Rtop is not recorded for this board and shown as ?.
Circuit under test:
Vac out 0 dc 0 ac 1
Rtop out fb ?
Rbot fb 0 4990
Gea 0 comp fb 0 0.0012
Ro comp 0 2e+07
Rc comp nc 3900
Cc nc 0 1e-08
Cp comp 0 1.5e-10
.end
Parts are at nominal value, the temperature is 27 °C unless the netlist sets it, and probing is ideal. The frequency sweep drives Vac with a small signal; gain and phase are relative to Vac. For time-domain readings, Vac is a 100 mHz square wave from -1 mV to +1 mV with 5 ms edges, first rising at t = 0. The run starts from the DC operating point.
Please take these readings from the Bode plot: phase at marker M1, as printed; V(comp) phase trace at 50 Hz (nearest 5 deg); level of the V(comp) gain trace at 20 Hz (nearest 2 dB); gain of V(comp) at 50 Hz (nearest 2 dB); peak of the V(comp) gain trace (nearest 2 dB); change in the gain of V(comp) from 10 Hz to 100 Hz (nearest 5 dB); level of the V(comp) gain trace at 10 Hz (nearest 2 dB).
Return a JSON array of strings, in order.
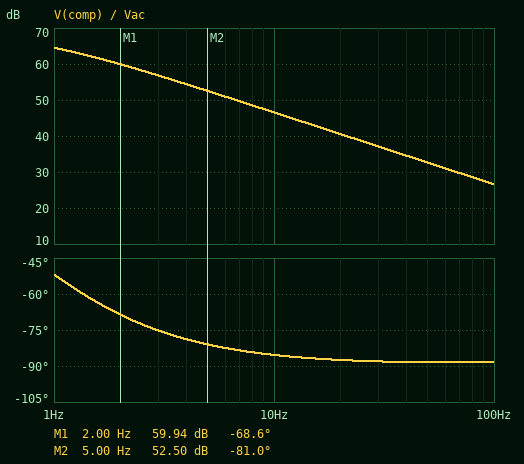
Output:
["-68.6 deg", "-90 deg", "40 dB", "32 dB", "64 dB", "-20 dB", "46 dB"]
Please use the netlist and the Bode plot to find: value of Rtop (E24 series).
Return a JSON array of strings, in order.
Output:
["39 kΩ"]
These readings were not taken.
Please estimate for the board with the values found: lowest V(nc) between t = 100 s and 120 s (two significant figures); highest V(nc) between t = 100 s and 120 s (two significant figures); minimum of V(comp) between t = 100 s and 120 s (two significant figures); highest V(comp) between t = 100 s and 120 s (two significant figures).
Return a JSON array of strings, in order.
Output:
["-2.7 V", "2.7 V", "-2.7 V", "2.7 V"]
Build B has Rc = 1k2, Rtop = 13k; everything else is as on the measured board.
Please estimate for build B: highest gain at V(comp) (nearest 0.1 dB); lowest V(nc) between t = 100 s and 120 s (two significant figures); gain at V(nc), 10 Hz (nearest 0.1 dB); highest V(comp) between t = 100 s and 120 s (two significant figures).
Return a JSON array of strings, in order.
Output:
["76.5 dB", "-6.7 V", "54.3 dB", "6.7 V"]
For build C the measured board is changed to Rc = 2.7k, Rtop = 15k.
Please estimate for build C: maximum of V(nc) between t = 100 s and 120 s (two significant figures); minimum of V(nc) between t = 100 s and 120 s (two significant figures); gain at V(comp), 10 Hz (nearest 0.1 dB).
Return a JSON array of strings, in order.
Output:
["6.0 V", "-6.0 V", "53.4 dB"]
